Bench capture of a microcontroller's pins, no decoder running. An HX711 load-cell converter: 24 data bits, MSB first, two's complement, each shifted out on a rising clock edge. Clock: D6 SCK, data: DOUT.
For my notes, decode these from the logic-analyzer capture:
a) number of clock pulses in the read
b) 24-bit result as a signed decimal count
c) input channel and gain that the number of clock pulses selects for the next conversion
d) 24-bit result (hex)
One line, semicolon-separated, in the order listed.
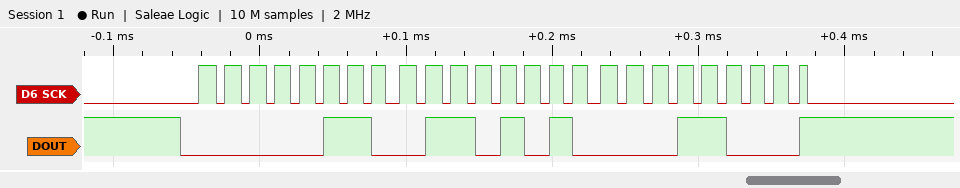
25; 420376; channel A, gain 128; 0x066A18
